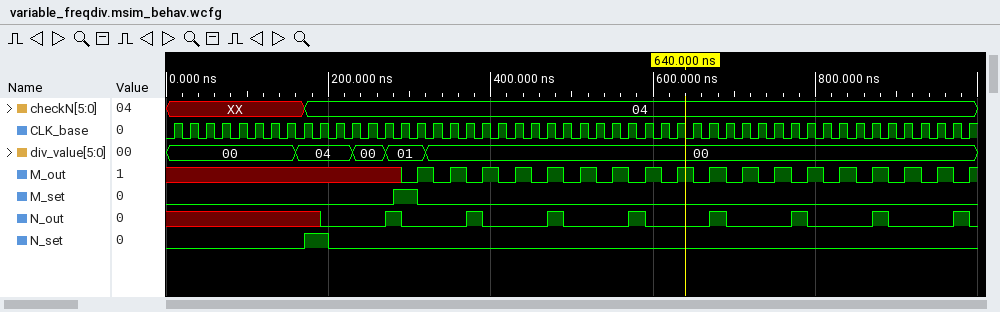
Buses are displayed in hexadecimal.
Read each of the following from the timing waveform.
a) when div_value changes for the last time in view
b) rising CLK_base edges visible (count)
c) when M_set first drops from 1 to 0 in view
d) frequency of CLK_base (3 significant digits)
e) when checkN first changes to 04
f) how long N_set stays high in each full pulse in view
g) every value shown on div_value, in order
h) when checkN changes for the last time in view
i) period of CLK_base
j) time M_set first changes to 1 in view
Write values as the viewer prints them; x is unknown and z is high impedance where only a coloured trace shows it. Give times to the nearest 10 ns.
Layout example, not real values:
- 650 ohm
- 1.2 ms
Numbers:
- 320 ns
- 50
- 310 ns
- 50.0 MHz
- 170 ns
- 30 ns
- 00, 04, 00, 01, 00
- 170 ns
- 20 ns
- 280 ns
